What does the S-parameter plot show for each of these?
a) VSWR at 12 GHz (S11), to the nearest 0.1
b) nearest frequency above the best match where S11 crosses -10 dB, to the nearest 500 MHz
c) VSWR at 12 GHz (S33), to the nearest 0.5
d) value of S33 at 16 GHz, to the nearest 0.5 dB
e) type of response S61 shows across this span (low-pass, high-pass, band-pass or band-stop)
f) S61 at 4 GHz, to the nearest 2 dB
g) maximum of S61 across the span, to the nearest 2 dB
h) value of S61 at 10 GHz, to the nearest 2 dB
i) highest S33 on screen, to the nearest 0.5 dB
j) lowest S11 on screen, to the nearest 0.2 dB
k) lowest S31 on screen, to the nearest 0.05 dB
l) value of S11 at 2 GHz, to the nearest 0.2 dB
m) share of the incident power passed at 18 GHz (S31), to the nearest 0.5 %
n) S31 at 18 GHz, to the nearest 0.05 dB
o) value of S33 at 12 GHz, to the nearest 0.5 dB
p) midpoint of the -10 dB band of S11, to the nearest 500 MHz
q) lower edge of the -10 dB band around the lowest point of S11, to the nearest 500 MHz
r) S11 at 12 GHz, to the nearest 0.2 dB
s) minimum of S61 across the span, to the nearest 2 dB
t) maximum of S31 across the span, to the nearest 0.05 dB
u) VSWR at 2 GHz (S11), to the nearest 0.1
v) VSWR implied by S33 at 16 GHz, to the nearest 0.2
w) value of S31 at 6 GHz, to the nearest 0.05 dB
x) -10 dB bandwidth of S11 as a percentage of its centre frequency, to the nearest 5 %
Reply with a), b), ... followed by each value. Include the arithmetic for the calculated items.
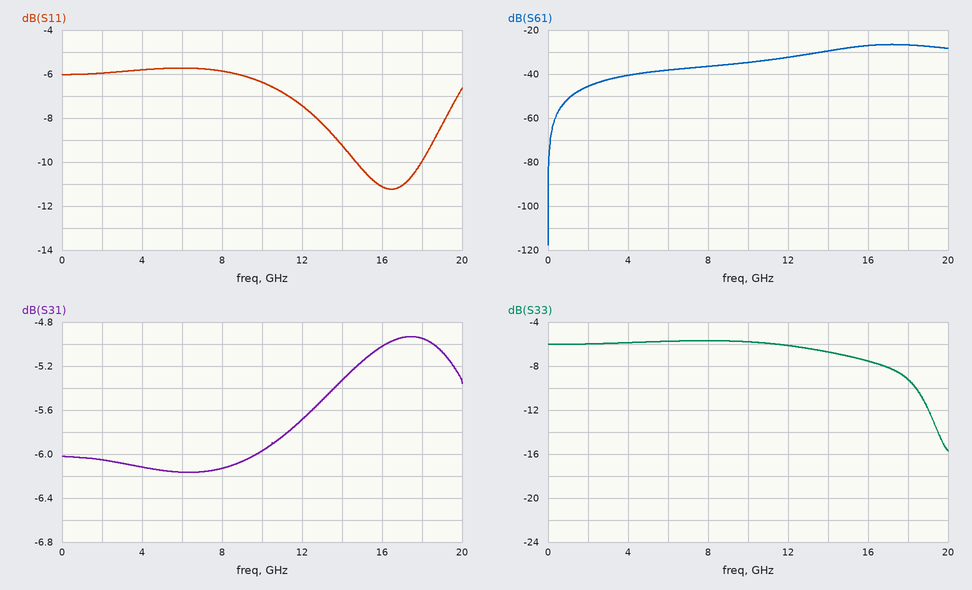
a) |Γ| = 10^(-7.4/20) = 0.4266; VSWR = (1 + 0.4266)/(1 − 0.4266) ≈ 2.5
b) 18.0 GHz
c) |Γ| = 10^(-6/20) = 0.5012; VSWR = (1 + 0.5012)/(1 − 0.5012) ≈ 3.0
d) -7.5 dB
e) high-pass
f) -40 dB
g) -26 dB
h) -34 dB
i) -5.5 dB
j) -11.2 dB
k) -6.15 dB
l) -6.0 dB
m) 10^(-4.95/10) ≈ 32.0 %
n) -4.95 dB
o) -6.0 dB
p) 16.5 GHz
q) 14.5 GHz
r) -7.4 dB
s) -118 dB
t) -4.95 dB
u) |Γ| = 10^(-6/20) = 0.5012; VSWR = (1 + 0.5012)/(1 − 0.5012) ≈ 3.0
v) |Γ| = 10^(-7.5/20) = 0.4217; VSWR = (1 + 0.4217)/(1 − 0.4217) ≈ 2.46, so 2.4 to the nearest 0.2
w) -6.15 dB
x) 3.5 GHz / 16.25 GHz ≈ 21.5 %, so 20 % to the nearest 5 %
